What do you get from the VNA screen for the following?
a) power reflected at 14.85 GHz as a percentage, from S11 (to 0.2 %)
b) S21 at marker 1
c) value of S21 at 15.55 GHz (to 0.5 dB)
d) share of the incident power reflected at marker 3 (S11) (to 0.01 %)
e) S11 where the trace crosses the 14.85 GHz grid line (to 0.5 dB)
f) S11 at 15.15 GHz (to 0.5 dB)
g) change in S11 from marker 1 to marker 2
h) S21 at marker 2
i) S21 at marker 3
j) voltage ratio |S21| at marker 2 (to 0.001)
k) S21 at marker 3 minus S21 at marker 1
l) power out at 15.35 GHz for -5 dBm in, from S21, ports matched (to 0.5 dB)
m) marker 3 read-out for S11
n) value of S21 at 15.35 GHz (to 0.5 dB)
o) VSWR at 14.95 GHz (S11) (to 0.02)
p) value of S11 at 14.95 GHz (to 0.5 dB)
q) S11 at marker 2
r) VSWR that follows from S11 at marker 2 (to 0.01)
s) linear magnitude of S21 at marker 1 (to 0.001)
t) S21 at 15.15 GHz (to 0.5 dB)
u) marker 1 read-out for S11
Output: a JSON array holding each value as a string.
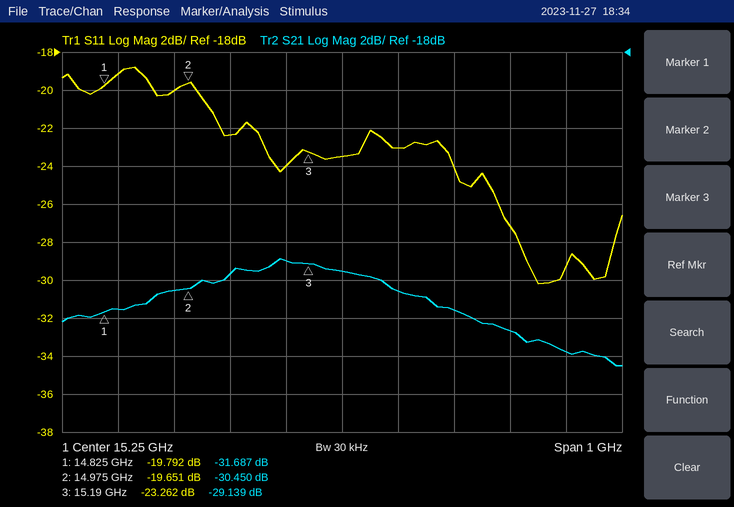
["1.2 %", "-31.687 dB", "-32.5 dB", "0.47 %", "-19.0 dB", "-24.0 dB", "0.141 dB", "-30.450 dB", "-29.139 dB", "0.030", "2.548 dB", "-35.5 dBm", "-23.262 dB", "-30.5 dB", "1.22", "-20.0 dB", "-19.651 dB", "1.23", "0.026", "-29.0 dB", "-19.792 dB"]
